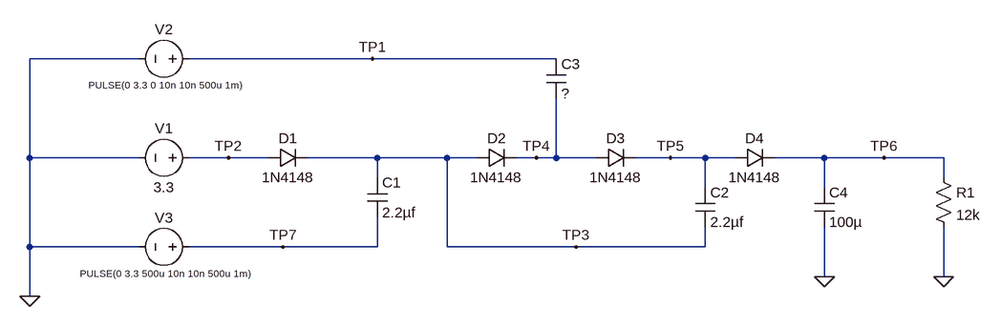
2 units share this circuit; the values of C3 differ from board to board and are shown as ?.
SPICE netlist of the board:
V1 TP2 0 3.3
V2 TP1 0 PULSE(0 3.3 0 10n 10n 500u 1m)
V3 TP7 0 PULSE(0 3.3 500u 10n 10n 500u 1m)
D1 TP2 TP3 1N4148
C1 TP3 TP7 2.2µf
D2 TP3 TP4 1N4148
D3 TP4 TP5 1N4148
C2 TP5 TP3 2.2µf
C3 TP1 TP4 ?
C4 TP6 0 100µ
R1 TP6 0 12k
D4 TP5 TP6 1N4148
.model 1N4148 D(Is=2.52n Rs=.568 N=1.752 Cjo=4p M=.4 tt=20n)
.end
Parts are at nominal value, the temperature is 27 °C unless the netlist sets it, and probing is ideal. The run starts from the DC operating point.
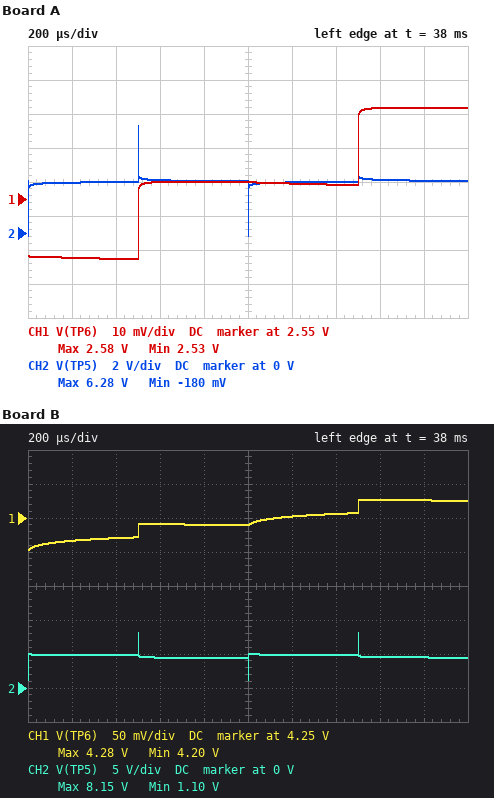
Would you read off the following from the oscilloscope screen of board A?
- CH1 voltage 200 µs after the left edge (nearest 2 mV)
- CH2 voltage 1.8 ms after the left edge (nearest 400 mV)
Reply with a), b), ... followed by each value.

a) 2.532 V
b) 3.2 V
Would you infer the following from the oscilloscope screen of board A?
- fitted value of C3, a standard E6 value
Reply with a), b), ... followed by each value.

a) 680 nF
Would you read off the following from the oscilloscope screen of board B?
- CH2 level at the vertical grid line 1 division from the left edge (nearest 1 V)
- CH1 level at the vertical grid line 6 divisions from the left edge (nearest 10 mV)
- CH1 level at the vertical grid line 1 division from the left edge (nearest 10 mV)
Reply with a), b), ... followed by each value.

a) 5 V
b) 4.25 V
c) 4.22 V
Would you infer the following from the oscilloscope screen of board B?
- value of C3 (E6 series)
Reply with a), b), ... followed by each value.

a) 6.8 µF
